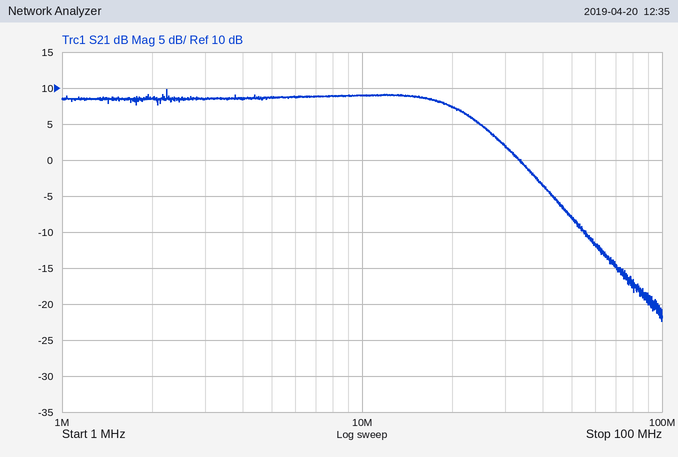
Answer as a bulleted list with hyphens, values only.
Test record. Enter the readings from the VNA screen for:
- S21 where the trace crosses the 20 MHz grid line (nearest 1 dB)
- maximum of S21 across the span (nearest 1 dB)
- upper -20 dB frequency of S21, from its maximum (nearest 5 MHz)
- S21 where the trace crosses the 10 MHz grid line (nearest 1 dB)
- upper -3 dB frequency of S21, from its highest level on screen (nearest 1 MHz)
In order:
- 7 dB
- 10 dB
- 55 MHz
- 9 dB
- 21 MHz
